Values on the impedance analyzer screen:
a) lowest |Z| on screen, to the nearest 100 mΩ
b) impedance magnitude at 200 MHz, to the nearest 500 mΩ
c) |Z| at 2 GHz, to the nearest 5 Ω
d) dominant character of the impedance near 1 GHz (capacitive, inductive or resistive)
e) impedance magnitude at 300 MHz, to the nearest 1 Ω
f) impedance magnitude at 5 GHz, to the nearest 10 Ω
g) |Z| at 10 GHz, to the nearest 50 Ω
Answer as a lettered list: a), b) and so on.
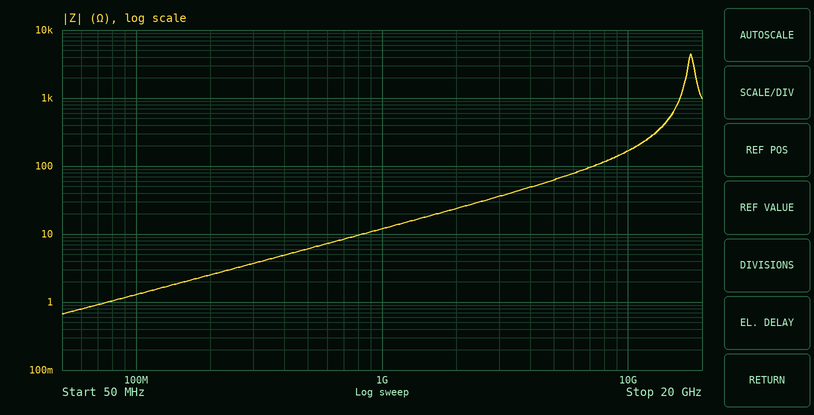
a) 700 mΩ
b) 2.5 Ω
c) 25 Ω
d) inductive
e) 4 Ω
f) 60 Ω
g) 150 Ω
